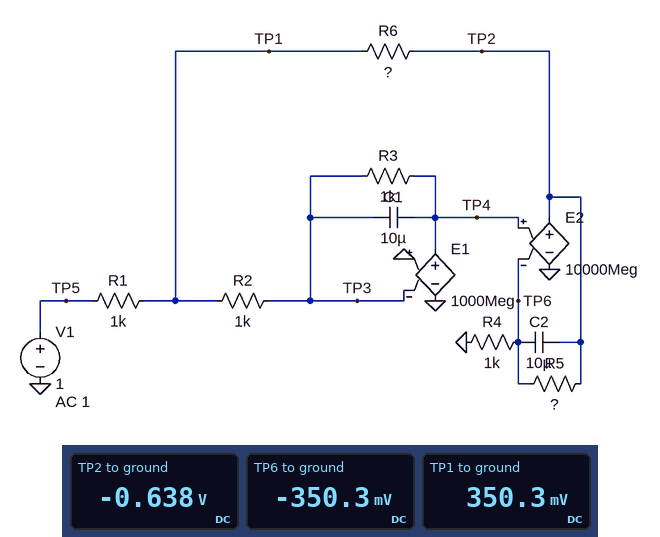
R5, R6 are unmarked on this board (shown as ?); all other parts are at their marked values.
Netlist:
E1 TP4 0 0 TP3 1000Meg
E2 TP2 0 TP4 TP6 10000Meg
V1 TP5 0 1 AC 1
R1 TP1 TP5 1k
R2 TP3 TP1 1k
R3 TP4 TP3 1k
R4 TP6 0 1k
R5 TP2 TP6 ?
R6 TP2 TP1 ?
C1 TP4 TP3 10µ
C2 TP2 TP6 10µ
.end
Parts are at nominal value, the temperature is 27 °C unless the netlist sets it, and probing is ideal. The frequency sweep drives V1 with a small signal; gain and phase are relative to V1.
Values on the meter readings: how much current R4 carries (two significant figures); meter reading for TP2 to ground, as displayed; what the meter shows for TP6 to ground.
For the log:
350 µA
-0.638 V
-350.3 mV
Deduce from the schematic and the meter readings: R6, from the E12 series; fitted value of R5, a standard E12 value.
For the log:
3.3 kΩ
820 Ω
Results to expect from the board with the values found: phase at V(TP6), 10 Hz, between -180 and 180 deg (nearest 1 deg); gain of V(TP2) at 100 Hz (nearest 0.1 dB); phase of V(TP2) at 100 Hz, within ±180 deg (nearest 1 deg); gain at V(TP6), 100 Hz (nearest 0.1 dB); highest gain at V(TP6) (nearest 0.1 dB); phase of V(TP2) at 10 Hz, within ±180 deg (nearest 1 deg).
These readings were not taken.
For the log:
154 deg
-23.0 dB
92 deg
-23.3 dB
-9.1 dB
143 deg
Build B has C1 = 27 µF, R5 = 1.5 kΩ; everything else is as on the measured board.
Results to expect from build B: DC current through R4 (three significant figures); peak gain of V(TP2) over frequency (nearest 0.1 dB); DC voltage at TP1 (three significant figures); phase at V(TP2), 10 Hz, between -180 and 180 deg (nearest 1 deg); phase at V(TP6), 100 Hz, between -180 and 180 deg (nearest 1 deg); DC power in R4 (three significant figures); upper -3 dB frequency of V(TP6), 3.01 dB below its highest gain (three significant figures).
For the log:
327 µA
-1.8 dB
327 mV
105 deg
94 deg
107 µW
8.86 Hz
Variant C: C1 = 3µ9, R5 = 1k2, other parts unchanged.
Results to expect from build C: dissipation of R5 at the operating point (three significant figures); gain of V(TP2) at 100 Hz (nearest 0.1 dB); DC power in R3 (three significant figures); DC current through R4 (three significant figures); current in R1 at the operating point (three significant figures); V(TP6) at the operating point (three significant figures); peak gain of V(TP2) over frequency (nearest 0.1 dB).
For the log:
136 µW
-15.5 dB
113 µW
337 µA
663 µA
-337 mV
-2.6 dB
